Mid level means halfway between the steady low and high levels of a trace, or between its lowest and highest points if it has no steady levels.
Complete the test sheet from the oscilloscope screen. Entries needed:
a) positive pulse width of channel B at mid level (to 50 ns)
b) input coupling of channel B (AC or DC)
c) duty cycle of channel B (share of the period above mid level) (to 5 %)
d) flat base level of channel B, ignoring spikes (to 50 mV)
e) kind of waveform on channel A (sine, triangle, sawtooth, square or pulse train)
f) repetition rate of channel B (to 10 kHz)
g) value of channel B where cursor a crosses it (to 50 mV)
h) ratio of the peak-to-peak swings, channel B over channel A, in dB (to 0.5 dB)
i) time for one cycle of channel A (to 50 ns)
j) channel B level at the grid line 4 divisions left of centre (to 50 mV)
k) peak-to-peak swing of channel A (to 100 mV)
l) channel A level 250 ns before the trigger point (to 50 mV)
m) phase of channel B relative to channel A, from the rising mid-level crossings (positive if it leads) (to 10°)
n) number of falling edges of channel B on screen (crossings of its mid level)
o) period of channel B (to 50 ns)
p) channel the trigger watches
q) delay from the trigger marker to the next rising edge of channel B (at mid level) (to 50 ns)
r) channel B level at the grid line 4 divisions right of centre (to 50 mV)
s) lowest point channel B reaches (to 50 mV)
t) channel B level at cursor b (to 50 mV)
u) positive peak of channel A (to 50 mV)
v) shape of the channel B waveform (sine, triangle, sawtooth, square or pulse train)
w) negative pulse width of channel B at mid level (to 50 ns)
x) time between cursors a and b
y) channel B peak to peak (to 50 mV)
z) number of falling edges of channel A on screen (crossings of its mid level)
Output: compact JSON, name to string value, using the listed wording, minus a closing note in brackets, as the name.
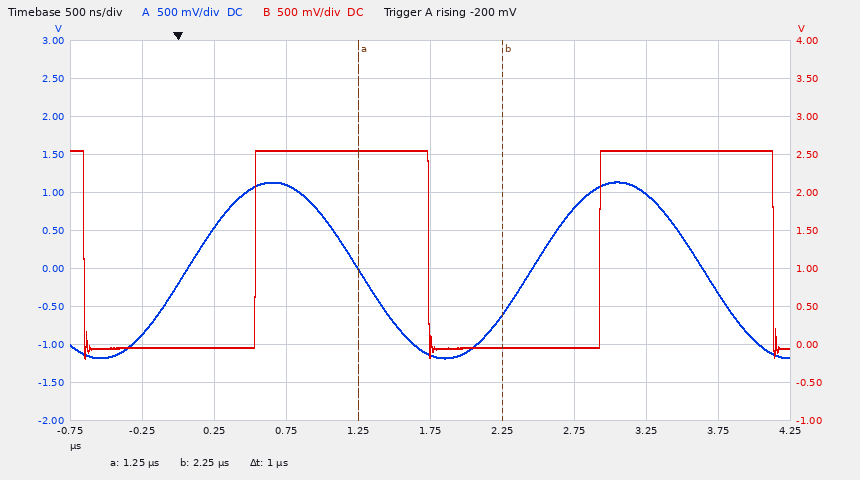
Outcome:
{"positive pulse width of channel B at mid level": "1.20 µs", "input coupling of channel B": "DC", "duty cycle of channel B (share of the period above mid level)": "50 %", "flat base level of channel B, ignoring spikes": "-50 mV", "kind of waveform on channel A": "sine", "repetition rate of channel B": "420 kHz", "value of channel B where cursor a crosses it": "2.55 V", "ratio of the peak-to-peak swings, channel B over channel A, in dB": "1.5 dB", "time for one cycle of channel A": "2.40 µs", "channel B level at the grid line 4 divisions left of centre": "-50 mV", "peak-to-peak swing of channel A": "2.30 V", "channel A level 250 ns before the trigger point": "-850 mV", "phase of channel B relative to channel A, from the rising mid-level crossings (positive if it leads)": "-70°", "number of falling edges of channel B on screen": "3", "period of channel B": "2.40 µs", "channel the trigger watches": "channel A", "delay from the trigger marker to the next rising edge of channel B (at mid level)": "550 ns", "channel B level at the grid line 4 divisions right of centre": "2.55 V", "lowest point channel B reaches": "-200 mV", "channel B level at cursor b": "-50 mV", "positive peak of channel A": "1.15 V", "shape of the channel B waveform": "square", "negative pulse width of channel B at mid level": "1.20 µs", "time between cursors a and b": "1 µs", "channel B peak to peak": "2.75 V", "number of falling edges of channel A on screen": "2"}
